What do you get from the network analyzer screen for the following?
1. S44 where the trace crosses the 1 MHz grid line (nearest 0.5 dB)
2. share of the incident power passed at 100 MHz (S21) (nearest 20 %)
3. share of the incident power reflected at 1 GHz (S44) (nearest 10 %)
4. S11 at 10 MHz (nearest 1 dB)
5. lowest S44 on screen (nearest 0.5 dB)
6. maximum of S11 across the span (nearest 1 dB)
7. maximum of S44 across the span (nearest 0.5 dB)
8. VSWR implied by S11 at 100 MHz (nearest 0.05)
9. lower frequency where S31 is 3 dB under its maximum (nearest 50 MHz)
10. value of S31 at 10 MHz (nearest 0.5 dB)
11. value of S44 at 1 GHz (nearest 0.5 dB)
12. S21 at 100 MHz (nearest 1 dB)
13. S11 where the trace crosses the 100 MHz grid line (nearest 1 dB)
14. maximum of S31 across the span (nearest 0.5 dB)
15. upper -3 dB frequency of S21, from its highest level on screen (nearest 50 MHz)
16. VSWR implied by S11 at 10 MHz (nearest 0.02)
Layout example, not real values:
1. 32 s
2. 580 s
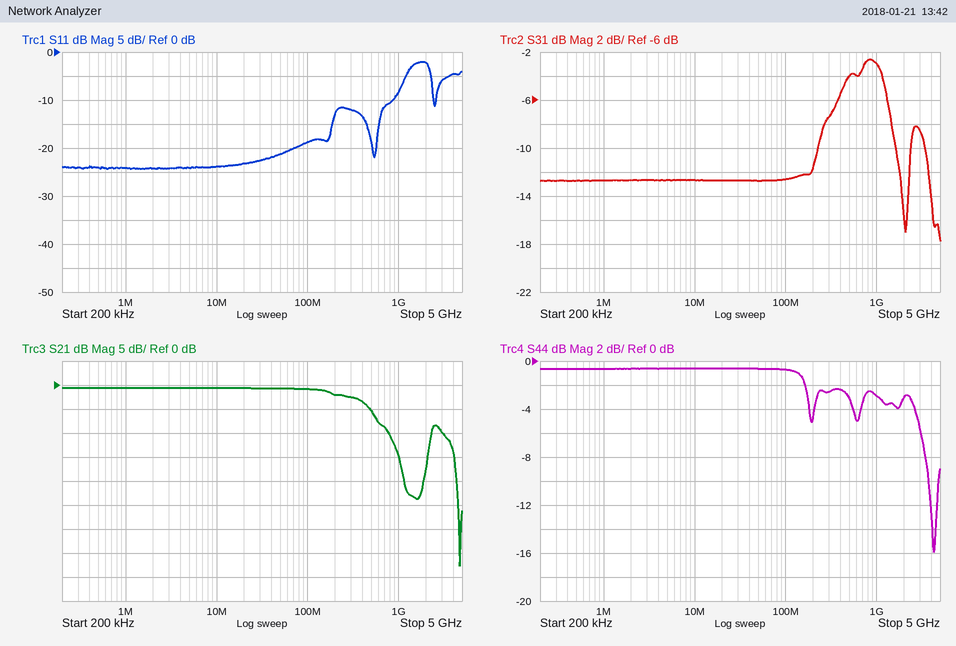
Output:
1. -0.5 dB
2. 80 %
3. 50 %
4. -24 dB
5. -16.0 dB
6. -2 dB
7. -0.5 dB
8. 1.25
9. 400 MHz
10. -12.5 dB
11. -3.0 dB
12. -1 dB
13. -19 dB
14. -2.5 dB
15. 400 MHz
16. 1.14
